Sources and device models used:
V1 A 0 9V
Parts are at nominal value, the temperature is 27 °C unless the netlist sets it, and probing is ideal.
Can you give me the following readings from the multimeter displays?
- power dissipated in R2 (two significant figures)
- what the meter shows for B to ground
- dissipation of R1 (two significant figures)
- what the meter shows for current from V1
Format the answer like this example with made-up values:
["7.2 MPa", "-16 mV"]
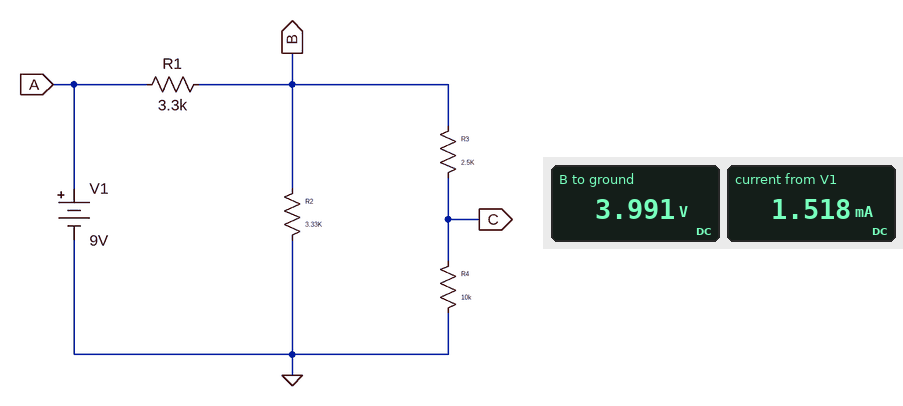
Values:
["4.8 mW", "3.991 V", "7.6 mW", "1.518 mA"]
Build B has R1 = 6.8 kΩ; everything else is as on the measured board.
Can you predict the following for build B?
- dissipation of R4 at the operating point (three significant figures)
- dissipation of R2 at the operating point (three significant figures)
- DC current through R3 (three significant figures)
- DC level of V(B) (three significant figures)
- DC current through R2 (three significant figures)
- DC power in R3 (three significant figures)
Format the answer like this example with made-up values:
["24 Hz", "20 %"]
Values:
["403 µW", "1.89 mW", "201 µA", "2.51 V", "754 µA", "101 µW"]
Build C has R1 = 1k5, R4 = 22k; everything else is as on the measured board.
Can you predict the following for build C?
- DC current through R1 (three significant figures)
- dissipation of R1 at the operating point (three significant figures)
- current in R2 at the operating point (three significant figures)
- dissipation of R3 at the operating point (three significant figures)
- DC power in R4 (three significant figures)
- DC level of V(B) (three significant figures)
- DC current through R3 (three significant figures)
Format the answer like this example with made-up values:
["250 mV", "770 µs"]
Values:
["2.03 mA", "6.19 mW", "1.79 mA", "148 µW", "1.30 mW", "5.95 V", "243 µA"]
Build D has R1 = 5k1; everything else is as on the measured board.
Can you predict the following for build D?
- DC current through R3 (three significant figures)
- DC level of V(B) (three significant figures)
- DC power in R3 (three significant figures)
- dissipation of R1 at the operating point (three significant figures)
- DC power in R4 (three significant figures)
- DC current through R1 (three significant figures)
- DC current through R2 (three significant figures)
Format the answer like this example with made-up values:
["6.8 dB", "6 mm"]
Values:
["245 µA", "3.06 V", "150 µW", "6.91 mW", "600 µW", "1.16 mA", "919 µA"]
